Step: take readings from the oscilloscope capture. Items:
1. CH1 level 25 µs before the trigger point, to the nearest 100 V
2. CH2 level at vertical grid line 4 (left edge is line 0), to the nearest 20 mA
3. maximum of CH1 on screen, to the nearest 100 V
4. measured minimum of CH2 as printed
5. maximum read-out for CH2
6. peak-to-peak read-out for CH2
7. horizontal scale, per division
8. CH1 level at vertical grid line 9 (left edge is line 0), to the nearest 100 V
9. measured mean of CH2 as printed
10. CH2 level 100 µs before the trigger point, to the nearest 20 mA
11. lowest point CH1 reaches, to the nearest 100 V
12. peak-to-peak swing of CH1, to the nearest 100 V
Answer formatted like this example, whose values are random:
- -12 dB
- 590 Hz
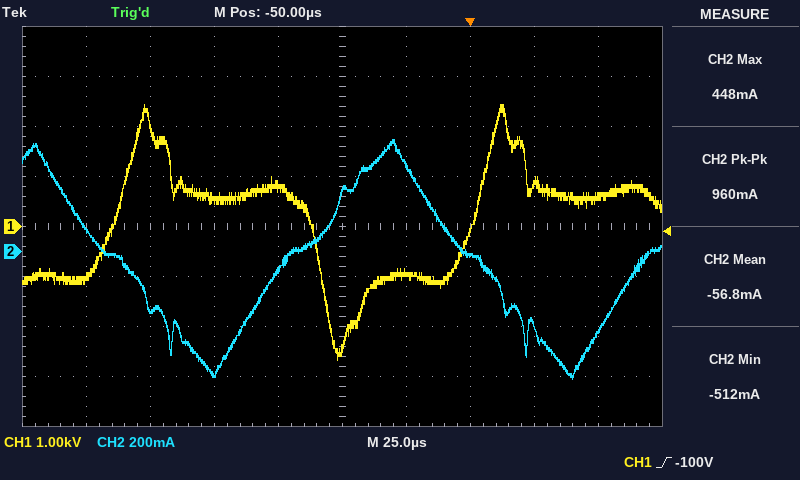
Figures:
- -900 V
- -80 mA
- 2.4 kV
- -512 mA
- 448 mA
- 960 mA
- 25 µs
- 600 V
- -56.8 mA
- -480 mA
- -2.7 kV
- 5.1 kV
